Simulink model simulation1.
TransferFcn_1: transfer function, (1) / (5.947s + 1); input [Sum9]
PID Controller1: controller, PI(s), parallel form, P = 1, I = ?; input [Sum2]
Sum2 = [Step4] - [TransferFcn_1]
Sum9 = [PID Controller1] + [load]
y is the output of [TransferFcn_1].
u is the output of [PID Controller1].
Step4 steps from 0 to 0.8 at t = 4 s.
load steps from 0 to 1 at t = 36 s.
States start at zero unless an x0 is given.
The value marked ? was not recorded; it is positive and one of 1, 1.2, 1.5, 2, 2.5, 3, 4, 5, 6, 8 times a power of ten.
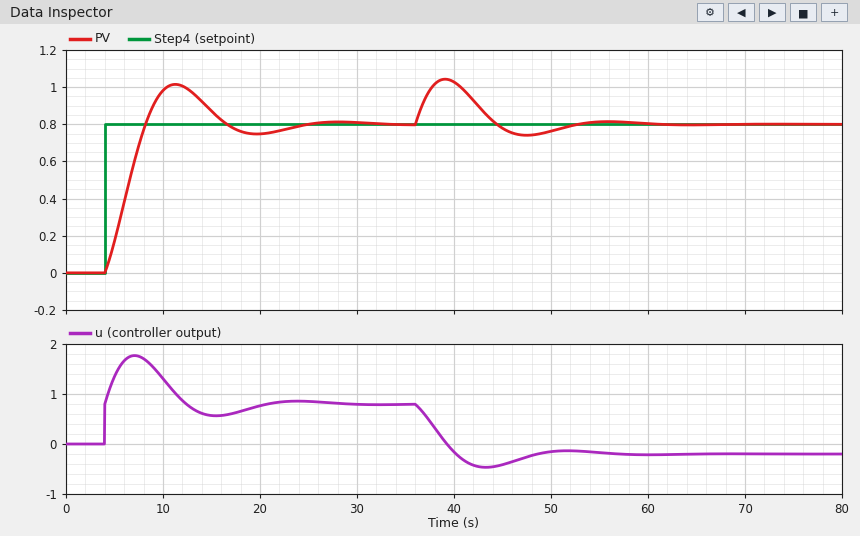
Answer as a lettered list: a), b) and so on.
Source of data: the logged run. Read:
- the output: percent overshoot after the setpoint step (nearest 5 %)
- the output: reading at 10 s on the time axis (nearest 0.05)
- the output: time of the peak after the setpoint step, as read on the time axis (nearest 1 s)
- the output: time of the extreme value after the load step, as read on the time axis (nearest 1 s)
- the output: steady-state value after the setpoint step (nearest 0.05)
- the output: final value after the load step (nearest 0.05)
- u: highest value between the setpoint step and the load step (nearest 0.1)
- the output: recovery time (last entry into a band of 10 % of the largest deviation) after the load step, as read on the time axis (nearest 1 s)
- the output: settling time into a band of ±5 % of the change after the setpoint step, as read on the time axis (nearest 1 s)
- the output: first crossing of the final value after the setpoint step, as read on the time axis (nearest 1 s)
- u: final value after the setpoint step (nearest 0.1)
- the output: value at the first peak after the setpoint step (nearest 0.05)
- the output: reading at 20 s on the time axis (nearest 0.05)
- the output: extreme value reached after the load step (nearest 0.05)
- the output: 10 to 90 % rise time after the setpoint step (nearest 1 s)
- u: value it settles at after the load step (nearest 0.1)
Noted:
a) 25 %
b) 1.00
c) 11 s
d) 39 s
e) 0.80
f) 0.80
g) 1.8
h) 51 s
i) 22 s
j) 8 s
k) 0.8
l) 1.00
m) 0.75
n) 1.05
o) 3 s
p) -0.2
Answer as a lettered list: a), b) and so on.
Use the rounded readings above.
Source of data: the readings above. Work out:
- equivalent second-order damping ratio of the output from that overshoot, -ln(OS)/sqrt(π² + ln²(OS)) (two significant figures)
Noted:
a) 0.40
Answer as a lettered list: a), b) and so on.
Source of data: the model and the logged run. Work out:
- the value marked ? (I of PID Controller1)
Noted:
a) 1
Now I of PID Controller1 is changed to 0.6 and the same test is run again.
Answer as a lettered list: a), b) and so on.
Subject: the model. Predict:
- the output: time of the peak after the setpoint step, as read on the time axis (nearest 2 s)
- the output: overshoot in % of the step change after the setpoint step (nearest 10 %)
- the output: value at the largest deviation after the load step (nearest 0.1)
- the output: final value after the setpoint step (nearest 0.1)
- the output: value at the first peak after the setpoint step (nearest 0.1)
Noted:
a) 14 s
b) 20 %
c) 1.1
d) 0.8
e) 0.9
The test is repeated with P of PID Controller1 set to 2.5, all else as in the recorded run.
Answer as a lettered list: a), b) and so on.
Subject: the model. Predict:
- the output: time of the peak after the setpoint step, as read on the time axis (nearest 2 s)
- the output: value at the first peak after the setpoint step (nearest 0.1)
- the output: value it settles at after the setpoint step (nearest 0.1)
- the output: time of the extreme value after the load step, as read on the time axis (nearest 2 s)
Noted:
a) 10 s
b) 0.9
c) 0.8
d) 38 s
